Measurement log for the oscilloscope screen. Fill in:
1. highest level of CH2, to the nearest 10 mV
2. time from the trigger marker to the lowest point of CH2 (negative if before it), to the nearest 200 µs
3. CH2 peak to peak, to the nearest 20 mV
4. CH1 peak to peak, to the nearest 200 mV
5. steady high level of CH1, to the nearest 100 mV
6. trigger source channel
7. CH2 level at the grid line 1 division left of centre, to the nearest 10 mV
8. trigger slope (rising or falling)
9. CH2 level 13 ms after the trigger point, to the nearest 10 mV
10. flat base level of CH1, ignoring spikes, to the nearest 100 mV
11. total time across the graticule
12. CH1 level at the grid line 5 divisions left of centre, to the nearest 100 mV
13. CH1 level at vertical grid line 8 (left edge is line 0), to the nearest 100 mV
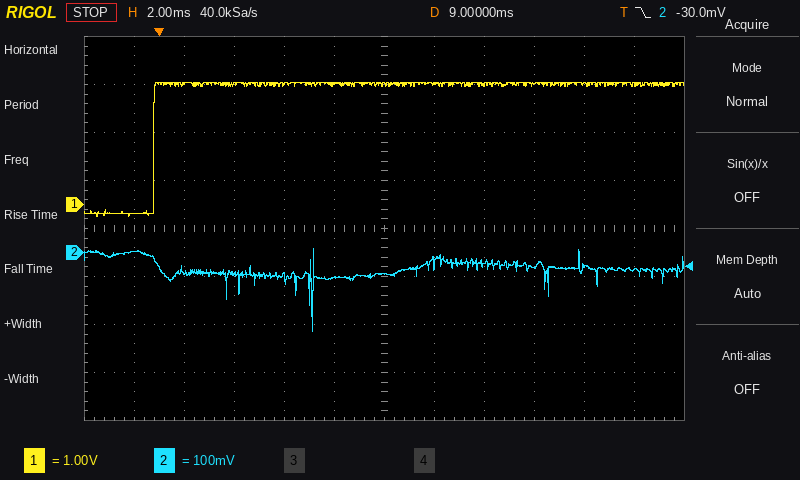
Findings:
10 mV
+6.2 ms
180 mV
2.8 V
2.5 V
CH2
-50 mV
falling
-20 mV
-200 mV
24 ms
-200 mV
2.5 V
